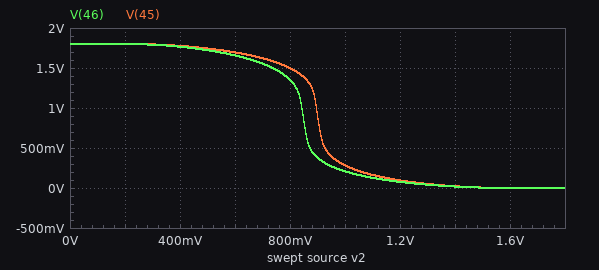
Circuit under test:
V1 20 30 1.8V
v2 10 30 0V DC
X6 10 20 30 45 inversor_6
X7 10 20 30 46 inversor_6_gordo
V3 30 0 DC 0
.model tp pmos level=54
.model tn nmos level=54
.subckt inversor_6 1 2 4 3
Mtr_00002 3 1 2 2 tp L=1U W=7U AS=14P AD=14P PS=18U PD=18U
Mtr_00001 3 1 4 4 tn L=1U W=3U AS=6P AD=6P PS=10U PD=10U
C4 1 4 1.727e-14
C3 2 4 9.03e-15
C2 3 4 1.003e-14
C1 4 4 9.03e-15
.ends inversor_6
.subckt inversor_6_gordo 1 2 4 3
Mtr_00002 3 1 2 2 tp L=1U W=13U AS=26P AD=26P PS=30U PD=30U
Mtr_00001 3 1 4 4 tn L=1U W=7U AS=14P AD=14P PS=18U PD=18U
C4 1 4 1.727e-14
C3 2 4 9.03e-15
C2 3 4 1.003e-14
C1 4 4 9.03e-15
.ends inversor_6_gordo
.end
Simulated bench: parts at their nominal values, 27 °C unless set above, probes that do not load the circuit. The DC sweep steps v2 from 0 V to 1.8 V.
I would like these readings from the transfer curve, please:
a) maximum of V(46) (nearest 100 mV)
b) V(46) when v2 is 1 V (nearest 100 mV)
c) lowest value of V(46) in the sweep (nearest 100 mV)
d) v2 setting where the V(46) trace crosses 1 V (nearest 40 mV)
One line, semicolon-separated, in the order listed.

1.8 V; 200 mV; 0 V; 840 mV
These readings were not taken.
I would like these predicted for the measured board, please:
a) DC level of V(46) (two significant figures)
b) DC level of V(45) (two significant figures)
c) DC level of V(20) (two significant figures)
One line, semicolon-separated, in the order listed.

1.8 V; 1.8 V; 1.8 V
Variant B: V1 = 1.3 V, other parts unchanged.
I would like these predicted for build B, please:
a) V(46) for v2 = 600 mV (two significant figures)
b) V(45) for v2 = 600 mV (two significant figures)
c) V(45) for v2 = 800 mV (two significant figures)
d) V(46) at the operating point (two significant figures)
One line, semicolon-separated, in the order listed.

920 mV; 1.1 V; 88 mV; 1.3 V
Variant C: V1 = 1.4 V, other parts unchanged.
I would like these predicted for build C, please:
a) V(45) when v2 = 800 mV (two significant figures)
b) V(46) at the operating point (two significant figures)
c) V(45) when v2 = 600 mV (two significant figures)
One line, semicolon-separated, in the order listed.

160 mV; 1.4 V; 1.2 V
